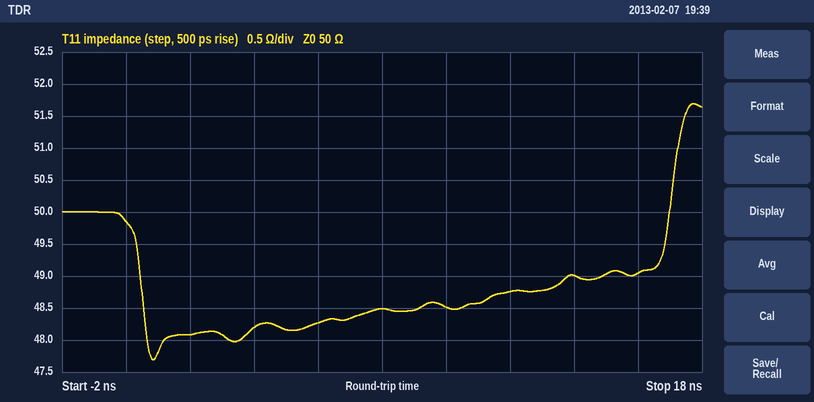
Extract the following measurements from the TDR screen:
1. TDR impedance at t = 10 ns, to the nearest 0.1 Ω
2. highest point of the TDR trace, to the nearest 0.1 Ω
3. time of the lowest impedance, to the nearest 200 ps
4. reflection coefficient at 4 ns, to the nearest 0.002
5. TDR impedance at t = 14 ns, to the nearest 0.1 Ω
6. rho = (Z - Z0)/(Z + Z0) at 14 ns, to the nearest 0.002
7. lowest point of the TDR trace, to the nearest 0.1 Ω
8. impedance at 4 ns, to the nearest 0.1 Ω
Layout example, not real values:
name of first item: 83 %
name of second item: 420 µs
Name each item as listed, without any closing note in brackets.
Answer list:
TDR impedance at t = 10 ns, to the nearest 0.1 Ω: 48.5 Ω
highest point of the TDR trace, to the nearest 0.1 Ω: 51.7 Ω
time of the lowest impedance, to the nearest 200 ps: 800 ps
reflection coefficient at 4 ns, to the nearest 0.002: -0.018
TDR impedance at t = 14 ns, to the nearest 0.1 Ω: 49.0 Ω
rho = (Z - Z0)/(Z + Z0) at 14 ns, to the nearest 0.002: -0.010
lowest point of the TDR trace, to the nearest 0.1 Ω: 47.7 Ω
impedance at 4 ns, to the nearest 0.1 Ω: 48.2 Ω
